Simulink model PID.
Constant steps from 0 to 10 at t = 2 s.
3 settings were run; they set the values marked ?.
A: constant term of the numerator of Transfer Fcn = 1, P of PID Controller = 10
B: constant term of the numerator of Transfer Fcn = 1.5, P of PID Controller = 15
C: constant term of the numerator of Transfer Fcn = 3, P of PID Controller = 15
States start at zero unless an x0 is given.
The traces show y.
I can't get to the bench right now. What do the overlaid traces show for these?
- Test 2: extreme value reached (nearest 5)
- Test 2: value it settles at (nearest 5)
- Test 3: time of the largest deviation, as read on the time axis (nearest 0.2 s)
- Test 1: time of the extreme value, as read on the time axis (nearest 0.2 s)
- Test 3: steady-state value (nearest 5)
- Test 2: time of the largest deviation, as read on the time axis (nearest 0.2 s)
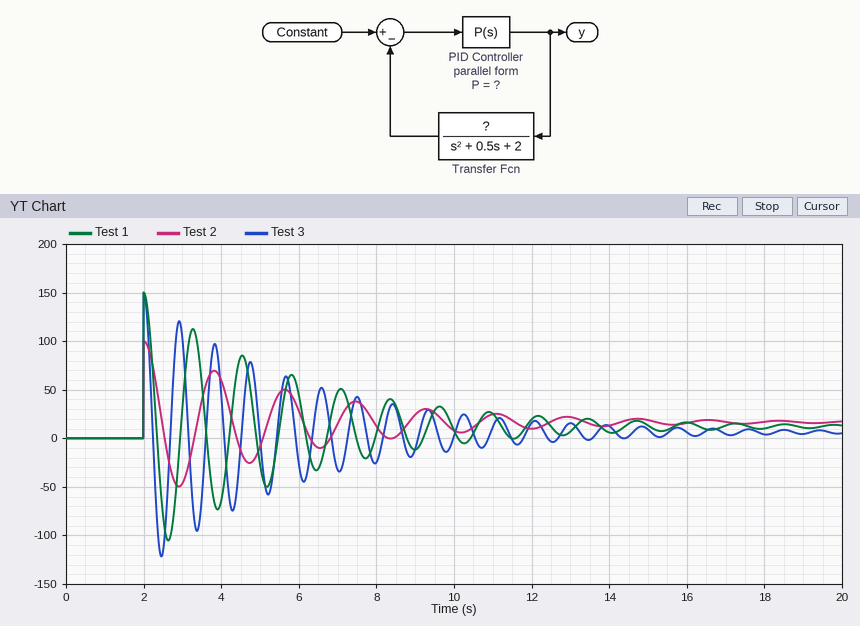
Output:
100
15
2.0 s
2.0 s
5
2.0 s
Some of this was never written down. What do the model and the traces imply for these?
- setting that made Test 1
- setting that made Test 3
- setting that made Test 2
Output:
B
C
A
